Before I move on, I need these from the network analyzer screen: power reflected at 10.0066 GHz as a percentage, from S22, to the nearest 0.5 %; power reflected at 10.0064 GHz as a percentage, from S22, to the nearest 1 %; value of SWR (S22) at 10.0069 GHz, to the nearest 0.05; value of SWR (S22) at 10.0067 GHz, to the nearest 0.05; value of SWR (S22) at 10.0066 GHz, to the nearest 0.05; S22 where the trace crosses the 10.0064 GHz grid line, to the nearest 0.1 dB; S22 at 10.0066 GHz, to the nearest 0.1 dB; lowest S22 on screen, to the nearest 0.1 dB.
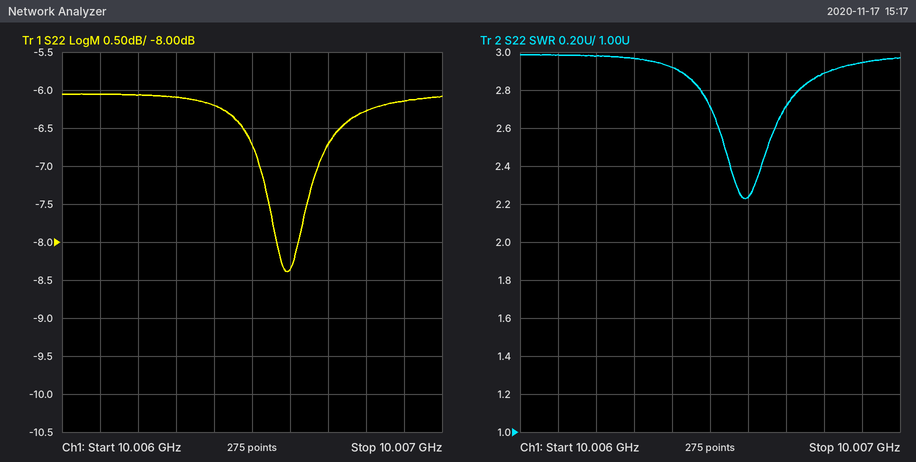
14.5 %
24 %
2.95
2.70
2.25
-6.2 dB
-8.4 dB
-8.4 dB
